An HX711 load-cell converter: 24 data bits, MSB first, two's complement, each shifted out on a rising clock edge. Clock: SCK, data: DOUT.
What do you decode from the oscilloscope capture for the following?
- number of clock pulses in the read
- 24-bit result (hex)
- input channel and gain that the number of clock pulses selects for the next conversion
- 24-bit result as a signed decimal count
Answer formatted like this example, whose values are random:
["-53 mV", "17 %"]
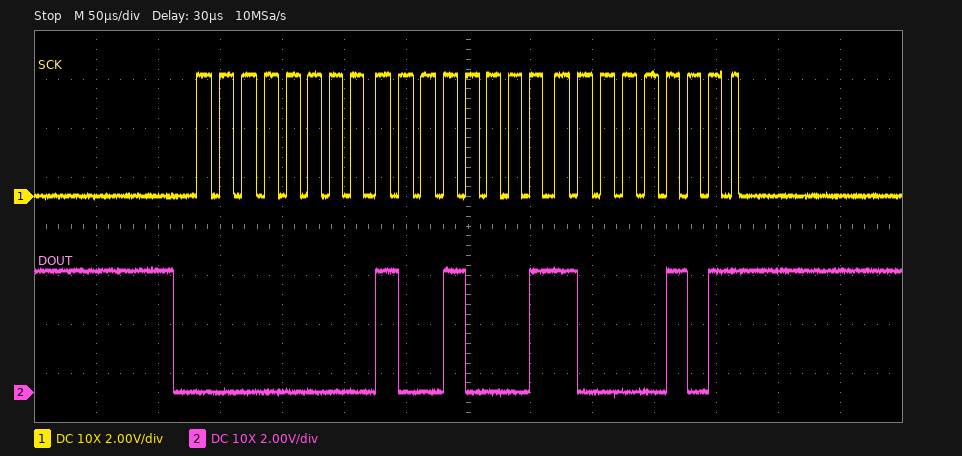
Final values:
["25", "0x009185", "channel A, gain 128", "37253"]
